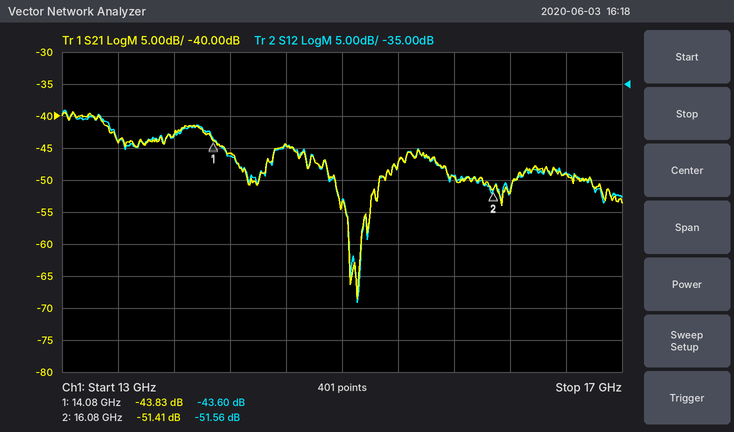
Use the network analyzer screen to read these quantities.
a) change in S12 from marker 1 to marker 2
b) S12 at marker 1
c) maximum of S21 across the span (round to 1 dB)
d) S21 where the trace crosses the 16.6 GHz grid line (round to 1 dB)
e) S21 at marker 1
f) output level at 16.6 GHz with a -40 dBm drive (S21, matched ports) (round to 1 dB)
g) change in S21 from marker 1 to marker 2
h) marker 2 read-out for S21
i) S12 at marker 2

-7.96 dB
-43.60 dB
-39 dB
-49 dB
-43.83 dB
-89 dBm
-7.58 dB
-51.41 dB
-51.56 dB
